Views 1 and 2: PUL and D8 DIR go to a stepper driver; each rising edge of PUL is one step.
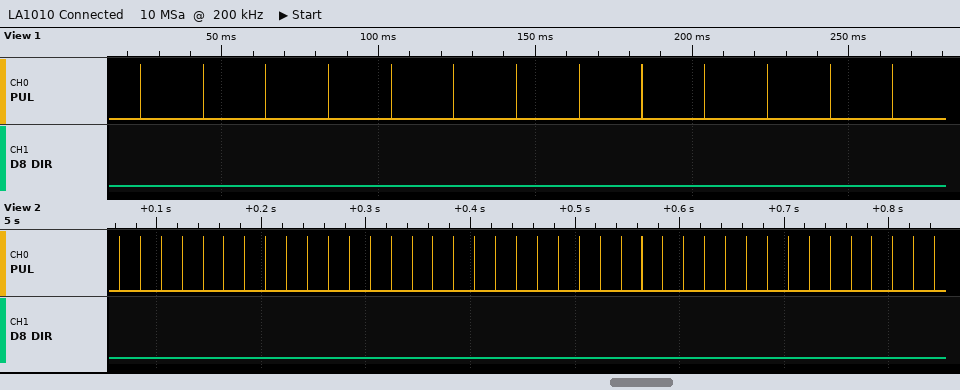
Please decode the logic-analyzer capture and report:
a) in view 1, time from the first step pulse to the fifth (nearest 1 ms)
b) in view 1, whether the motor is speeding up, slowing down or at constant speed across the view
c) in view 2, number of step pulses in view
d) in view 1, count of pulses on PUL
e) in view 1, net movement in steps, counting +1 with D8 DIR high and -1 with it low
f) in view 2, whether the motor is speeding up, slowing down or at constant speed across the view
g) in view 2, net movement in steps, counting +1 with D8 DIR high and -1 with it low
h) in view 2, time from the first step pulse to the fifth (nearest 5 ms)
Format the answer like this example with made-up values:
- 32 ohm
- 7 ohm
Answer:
- 80 ms
- constant speed
- 40
- 13
- -13
- constant speed
- -40
- 80 ms
